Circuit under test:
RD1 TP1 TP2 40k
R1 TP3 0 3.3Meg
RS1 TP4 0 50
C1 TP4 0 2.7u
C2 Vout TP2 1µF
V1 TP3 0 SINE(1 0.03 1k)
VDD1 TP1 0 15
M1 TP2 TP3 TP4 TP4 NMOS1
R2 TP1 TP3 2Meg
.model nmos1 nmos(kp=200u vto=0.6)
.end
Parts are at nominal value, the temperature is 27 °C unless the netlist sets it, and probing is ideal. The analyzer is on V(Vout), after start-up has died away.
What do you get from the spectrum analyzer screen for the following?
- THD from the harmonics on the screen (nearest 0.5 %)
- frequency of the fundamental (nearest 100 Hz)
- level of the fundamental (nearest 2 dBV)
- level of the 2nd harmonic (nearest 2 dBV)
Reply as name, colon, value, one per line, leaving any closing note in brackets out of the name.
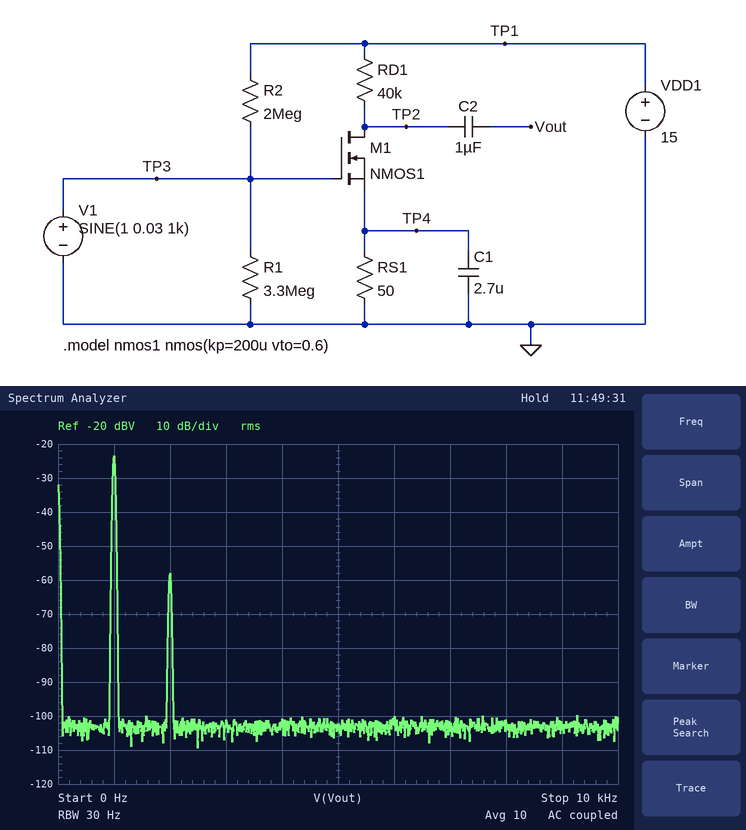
THD from the harmonics on the screen: 2.0 %
frequency of the fundamental: 1.0 kHz
level of the fundamental: -24 dBV
level of the 2nd harmonic: -58 dBV
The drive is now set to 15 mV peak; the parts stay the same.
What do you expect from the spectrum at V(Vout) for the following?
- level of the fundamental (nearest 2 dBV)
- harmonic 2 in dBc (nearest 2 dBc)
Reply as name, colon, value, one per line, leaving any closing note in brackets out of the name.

level of the fundamental: -30 dBV
harmonic 2 in dBc: -40 dBc
